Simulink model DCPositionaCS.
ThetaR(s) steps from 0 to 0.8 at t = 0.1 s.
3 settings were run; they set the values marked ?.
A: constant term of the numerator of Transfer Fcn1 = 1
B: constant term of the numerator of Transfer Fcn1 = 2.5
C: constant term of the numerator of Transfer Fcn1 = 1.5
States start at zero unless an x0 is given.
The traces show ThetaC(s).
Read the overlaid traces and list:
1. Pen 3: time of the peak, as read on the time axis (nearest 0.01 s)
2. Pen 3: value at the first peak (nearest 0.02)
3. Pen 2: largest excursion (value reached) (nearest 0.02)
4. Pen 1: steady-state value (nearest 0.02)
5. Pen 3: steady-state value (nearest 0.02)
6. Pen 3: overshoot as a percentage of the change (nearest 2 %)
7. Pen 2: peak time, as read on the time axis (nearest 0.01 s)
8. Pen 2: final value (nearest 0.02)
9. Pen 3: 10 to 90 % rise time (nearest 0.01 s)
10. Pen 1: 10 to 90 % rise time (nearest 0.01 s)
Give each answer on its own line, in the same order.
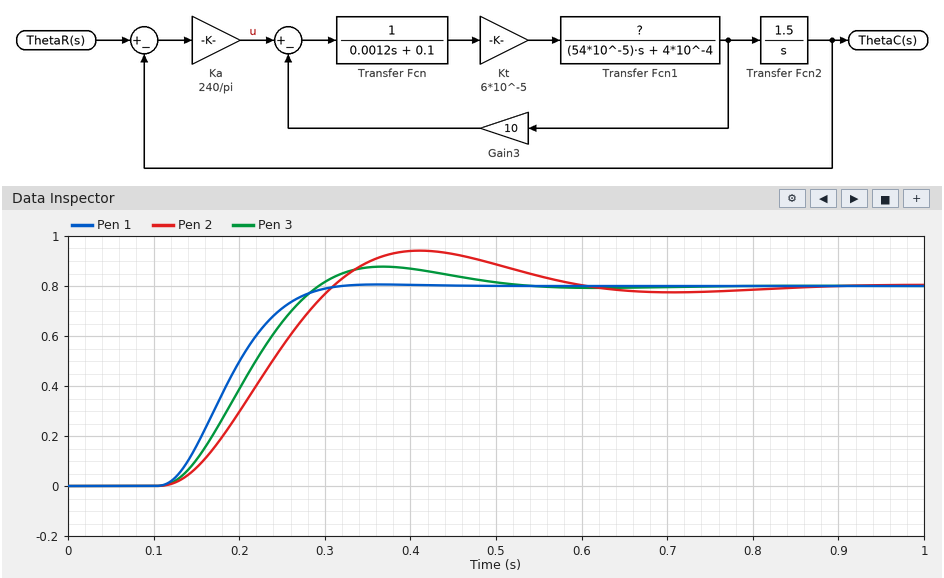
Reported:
0.37 s
0.88
0.94
0.80
0.80
10 %
0.41 s
0.80
0.12 s
0.12 s
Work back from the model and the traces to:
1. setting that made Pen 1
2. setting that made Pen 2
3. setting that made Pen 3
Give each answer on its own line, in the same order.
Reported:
B
A
C
